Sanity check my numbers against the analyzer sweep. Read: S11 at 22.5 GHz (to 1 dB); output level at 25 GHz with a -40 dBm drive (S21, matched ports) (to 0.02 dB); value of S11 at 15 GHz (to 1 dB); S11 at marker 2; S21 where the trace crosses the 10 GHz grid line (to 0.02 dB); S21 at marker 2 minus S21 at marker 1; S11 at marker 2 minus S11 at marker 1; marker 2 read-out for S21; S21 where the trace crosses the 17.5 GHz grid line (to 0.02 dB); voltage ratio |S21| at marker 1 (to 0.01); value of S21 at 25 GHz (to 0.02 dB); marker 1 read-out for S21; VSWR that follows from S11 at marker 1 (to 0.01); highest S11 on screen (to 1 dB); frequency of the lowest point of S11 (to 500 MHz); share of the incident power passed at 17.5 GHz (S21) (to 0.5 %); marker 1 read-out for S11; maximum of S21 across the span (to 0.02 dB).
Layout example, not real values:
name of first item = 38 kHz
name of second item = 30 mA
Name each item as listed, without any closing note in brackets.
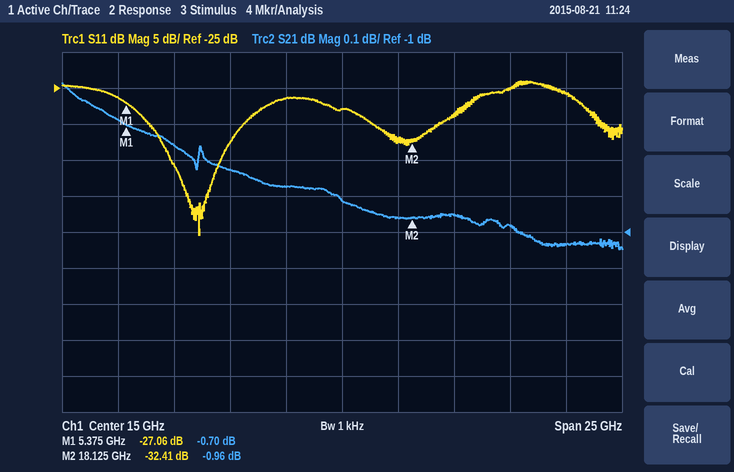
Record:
S11 at 22.5 GHz = -25 dB
output level at 25 GHz with a -40 dBm drive (S21, matched ports) = -41.04 dBm
value of S11 at 15 GHz = -28 dB
S11 at marker 2 = -32.41 dB
S21 where the trace crosses the 10 GHz grid line = -0.82 dB
S21 at marker 2 minus S21 at marker 1 = -0.26 dB
S11 at marker 2 minus S11 at marker 1 = -5.35 dB
marker 2 read-out for S21 = -0.96 dB
S21 where the trace crosses the 17.5 GHz grid line = -0.96 dB
voltage ratio |S21| at marker 1 = 0.92
value of S21 at 25 GHz = -1.04 dB
marker 1 read-out for S21 = -0.70 dB
VSWR that follows from S11 at marker 1 = 1.09
highest S11 on screen = -24 dB
frequency of the lowest point of S11 = 8.5 GHz
share of the incident power passed at 17.5 GHz (S21) = 80.0 %
marker 1 read-out for S11 = -27.06 dB
maximum of S21 across the span = -0.58 dB
